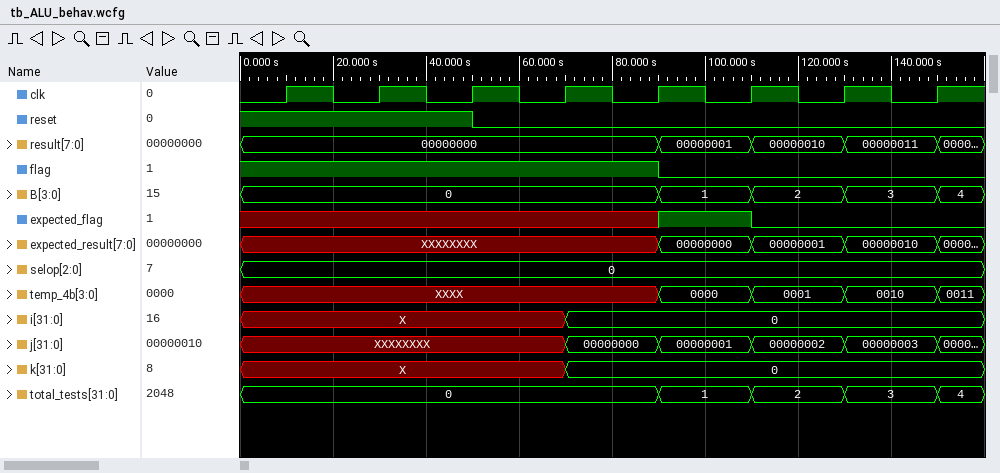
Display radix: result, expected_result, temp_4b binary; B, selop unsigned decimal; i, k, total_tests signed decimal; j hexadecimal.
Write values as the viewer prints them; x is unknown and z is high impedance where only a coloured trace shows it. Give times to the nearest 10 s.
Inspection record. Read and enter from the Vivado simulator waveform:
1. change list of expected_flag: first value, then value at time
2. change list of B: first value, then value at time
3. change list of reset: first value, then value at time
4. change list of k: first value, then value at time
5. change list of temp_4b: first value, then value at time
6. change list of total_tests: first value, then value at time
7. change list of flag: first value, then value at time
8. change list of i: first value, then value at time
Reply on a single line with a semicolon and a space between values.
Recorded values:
x, 1 at 90 s, 0 at 110 s; 0, 1 at 90 s, 2 at 110 s, 3 at 130 s, 4 at 150 s; 1, 0 at 50 s; X, 0 at 70 s; XXXX, 0000 at 90 s, 0001 at 110 s, 0010 at 130 s, 0011 at 150 s; 0, 1 at 90 s, 2 at 110 s, 3 at 130 s, 4 at 150 s; 1, 0 at 90 s; X, 0 at 70 s
